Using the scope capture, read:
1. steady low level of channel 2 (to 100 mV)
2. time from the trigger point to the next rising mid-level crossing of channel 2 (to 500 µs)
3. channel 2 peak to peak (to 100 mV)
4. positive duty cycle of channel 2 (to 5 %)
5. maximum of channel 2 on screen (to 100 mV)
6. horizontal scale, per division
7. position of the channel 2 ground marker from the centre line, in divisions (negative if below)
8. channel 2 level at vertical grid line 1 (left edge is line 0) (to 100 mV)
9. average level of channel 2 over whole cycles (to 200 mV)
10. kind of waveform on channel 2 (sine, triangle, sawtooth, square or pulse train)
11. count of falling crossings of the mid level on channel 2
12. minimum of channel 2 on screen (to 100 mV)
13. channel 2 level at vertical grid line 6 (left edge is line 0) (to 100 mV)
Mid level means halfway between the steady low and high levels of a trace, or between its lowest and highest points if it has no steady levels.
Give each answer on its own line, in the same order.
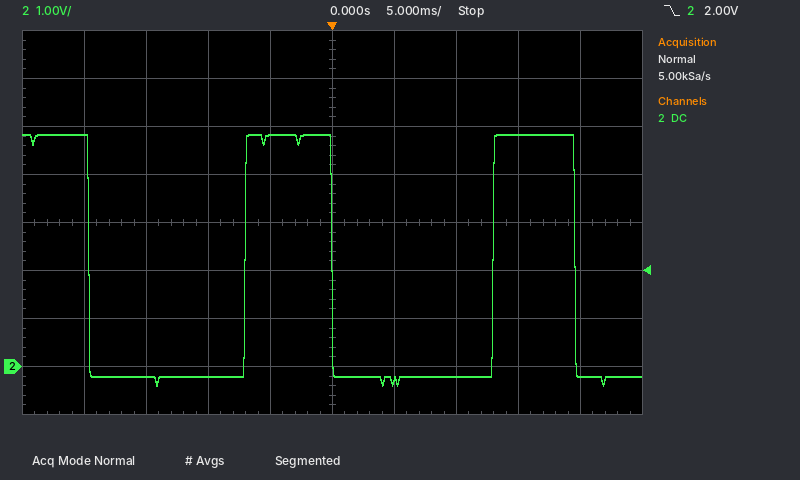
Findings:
-200 mV
13.0 ms
5.2 V
35 %
4.8 V
5 ms
-3.0 div
4.8 V
1.6 V
pulse train
3
-400 mV
-300 mV
